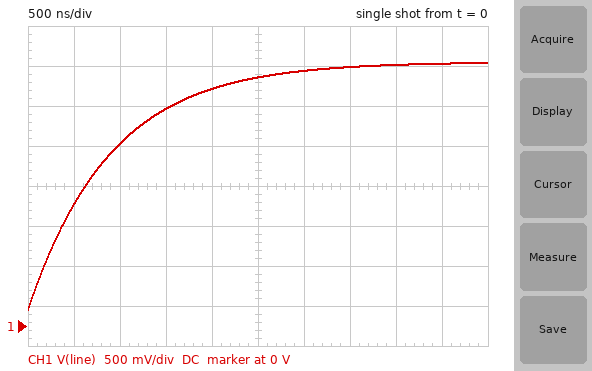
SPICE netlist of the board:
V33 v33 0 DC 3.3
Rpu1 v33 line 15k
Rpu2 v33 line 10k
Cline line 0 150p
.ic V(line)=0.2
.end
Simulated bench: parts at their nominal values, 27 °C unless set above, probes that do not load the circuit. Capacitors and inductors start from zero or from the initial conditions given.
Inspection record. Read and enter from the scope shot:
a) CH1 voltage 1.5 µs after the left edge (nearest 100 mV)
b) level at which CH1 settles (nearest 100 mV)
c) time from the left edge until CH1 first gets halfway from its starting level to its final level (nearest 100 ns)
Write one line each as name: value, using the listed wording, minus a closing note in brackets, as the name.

CH1 voltage 1.5 µs after the left edge: 2.7 V
level at which CH1 settles: 3.3 V
time from the left edge until CH1 first gets halfway from its starting level to its final level: 600 ns
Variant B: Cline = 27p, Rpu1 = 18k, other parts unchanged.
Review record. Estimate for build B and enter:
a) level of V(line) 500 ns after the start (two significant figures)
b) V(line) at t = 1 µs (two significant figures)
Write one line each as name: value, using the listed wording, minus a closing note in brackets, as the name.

level of V(line) 500 ns after the start: 3.1 V
V(line) at t = 1 µs: 3.3 V
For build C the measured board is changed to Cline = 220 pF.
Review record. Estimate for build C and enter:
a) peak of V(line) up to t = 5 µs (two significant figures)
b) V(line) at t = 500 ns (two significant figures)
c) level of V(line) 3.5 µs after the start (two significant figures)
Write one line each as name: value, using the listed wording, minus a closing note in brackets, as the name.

peak of V(line) up to t = 5 µs: 3.2 V
V(line) at t = 500 ns: 1.2 V
level of V(line) 3.5 µs after the start: 3.1 V
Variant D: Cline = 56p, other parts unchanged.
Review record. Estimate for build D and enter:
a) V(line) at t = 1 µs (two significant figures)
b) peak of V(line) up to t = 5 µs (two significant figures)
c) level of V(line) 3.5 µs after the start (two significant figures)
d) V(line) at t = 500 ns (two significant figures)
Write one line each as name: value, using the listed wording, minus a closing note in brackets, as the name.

V(line) at t = 1 µs: 3.1 V
peak of V(line) up to t = 5 µs: 3.3 V
level of V(line) 3.5 µs after the start: 3.3 V
V(line) at t = 500 ns: 2.6 V
